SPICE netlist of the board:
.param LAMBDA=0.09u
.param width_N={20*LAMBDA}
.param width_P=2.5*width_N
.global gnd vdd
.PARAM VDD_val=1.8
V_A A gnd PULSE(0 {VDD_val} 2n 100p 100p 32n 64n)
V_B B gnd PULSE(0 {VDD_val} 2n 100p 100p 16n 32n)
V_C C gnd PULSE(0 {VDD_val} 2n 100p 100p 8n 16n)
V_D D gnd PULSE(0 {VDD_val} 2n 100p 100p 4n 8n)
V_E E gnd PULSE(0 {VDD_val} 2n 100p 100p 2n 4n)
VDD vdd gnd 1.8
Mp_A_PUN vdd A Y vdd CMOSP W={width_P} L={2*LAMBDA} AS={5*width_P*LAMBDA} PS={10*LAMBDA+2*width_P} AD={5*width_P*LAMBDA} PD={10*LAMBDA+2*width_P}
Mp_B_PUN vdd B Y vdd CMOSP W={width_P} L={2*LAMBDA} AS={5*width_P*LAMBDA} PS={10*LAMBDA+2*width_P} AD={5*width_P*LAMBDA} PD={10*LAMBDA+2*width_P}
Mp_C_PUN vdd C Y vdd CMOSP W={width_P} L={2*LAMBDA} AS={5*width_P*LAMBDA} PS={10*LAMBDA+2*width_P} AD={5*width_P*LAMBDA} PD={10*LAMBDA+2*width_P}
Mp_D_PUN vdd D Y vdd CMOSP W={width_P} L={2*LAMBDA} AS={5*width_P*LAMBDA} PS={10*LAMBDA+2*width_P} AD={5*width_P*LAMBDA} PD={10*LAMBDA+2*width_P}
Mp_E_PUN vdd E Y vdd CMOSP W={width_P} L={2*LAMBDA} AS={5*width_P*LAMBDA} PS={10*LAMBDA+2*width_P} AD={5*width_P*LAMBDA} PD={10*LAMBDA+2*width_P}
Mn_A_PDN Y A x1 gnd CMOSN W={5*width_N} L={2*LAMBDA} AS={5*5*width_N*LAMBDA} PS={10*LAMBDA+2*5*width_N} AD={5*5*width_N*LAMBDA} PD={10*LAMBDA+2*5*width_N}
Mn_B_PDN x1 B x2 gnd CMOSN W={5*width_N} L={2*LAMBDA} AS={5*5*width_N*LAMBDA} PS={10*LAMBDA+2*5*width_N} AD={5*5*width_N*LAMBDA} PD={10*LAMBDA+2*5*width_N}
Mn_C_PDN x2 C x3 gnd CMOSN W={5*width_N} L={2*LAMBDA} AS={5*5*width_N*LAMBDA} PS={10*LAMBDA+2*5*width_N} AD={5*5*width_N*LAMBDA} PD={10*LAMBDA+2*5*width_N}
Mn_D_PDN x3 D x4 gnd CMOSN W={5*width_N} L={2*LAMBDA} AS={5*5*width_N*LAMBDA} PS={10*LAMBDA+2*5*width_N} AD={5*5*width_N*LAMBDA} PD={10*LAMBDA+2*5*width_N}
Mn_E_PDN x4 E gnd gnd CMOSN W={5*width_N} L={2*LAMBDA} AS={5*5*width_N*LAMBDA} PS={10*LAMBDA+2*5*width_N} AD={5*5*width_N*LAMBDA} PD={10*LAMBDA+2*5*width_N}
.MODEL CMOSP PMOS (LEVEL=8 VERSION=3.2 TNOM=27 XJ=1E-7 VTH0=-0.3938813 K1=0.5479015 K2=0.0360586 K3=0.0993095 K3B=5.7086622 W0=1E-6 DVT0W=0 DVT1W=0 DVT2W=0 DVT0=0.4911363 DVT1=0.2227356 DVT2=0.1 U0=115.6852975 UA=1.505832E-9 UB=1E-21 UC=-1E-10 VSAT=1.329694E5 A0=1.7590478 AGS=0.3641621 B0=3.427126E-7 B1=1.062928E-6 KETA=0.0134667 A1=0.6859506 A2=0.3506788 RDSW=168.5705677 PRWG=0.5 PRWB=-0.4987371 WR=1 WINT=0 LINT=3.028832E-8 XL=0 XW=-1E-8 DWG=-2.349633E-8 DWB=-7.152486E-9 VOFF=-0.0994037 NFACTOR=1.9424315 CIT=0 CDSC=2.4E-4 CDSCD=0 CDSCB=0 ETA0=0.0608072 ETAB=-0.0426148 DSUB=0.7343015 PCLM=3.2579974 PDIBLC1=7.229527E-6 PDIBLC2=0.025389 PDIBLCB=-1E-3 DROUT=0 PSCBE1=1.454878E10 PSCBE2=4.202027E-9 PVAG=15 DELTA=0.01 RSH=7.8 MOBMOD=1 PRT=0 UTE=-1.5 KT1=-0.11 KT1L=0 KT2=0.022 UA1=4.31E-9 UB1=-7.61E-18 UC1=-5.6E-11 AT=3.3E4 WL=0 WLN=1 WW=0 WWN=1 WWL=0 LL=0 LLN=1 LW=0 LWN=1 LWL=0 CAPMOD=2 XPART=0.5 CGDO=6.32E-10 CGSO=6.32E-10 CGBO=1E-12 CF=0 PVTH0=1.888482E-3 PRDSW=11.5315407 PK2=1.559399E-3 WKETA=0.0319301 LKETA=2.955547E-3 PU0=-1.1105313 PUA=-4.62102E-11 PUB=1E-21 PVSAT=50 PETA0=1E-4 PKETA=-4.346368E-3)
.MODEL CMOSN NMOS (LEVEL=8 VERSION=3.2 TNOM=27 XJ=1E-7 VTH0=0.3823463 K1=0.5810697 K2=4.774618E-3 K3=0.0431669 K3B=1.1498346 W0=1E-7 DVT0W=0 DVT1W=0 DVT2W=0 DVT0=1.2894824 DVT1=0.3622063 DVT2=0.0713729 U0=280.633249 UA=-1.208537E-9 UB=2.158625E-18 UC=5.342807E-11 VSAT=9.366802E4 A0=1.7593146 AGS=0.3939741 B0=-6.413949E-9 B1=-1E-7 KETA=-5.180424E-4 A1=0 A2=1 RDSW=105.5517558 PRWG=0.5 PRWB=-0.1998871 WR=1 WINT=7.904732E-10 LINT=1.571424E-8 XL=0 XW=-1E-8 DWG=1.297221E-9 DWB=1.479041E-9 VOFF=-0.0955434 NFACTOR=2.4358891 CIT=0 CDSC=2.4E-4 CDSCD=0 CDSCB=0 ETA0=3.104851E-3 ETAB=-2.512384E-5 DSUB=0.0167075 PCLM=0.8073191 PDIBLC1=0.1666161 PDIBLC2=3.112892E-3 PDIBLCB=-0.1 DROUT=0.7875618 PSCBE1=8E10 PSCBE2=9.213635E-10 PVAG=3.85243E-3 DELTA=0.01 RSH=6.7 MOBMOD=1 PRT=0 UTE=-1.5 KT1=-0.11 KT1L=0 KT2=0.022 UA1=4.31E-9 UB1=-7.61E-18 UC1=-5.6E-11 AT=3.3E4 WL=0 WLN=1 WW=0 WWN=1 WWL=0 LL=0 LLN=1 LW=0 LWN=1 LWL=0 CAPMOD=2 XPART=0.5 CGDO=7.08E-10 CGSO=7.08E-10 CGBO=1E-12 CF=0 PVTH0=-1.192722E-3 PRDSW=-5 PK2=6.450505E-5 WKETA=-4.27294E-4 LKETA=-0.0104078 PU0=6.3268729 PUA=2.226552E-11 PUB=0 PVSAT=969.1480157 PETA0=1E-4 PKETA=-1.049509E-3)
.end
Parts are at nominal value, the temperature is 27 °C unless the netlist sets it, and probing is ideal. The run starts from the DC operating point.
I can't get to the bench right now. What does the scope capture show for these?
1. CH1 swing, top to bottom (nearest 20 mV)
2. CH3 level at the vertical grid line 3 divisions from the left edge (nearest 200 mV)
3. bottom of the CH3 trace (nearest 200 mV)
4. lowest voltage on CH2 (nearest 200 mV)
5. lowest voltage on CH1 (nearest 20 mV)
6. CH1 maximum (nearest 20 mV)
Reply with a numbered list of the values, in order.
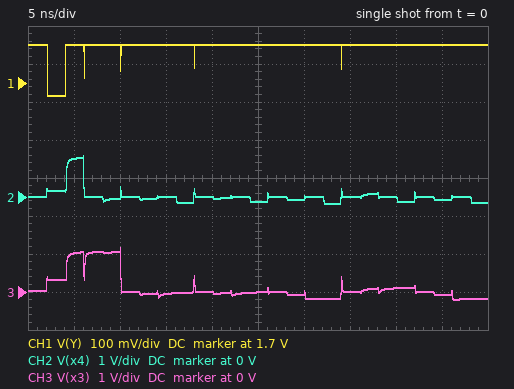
1. 140 mV
2. 0 V
3. -200 mV
4. -200 mV
5. 1.66 V
6. 1.80 V
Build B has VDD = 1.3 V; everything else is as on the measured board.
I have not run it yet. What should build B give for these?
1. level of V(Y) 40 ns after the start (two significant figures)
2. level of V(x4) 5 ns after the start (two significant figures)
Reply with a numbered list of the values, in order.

1. 1.3 V
2. 980 mV
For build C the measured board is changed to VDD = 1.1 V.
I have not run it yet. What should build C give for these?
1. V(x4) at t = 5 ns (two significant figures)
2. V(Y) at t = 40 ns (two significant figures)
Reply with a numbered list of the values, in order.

1. 970 mV
2. 1.1 V
